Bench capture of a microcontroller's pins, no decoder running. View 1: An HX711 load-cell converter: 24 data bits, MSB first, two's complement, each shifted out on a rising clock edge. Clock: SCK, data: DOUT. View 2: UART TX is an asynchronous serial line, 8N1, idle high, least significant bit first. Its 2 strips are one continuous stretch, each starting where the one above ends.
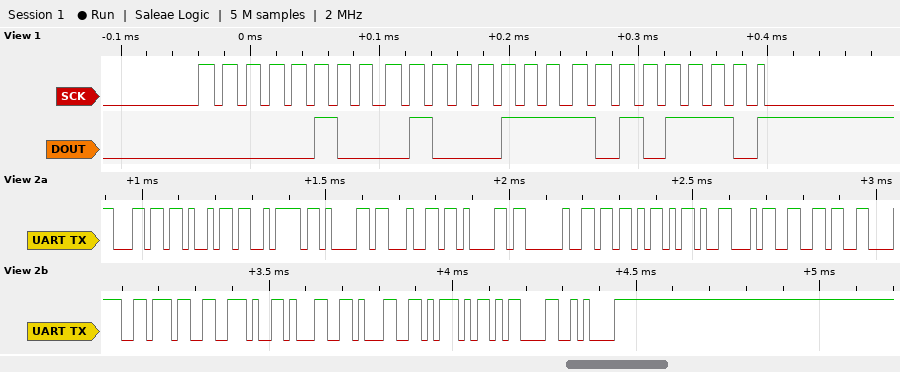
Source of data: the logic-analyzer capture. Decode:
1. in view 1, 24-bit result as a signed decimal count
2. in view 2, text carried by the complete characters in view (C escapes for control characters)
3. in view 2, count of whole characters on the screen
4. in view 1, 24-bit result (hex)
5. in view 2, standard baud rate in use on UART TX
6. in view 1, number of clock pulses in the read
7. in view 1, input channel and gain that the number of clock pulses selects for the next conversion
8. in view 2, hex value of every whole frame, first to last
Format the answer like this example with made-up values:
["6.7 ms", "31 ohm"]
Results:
["280494", "\"lizada [-4687.11]\\r\\n\"", "19", "0x0447AE", "57600 baud", "25", "channel A, gain 128", "6C 69 7A 61 64 61 20 5B 2D 34 36 38 37 2E 31 31 5D 0D 0A"]
